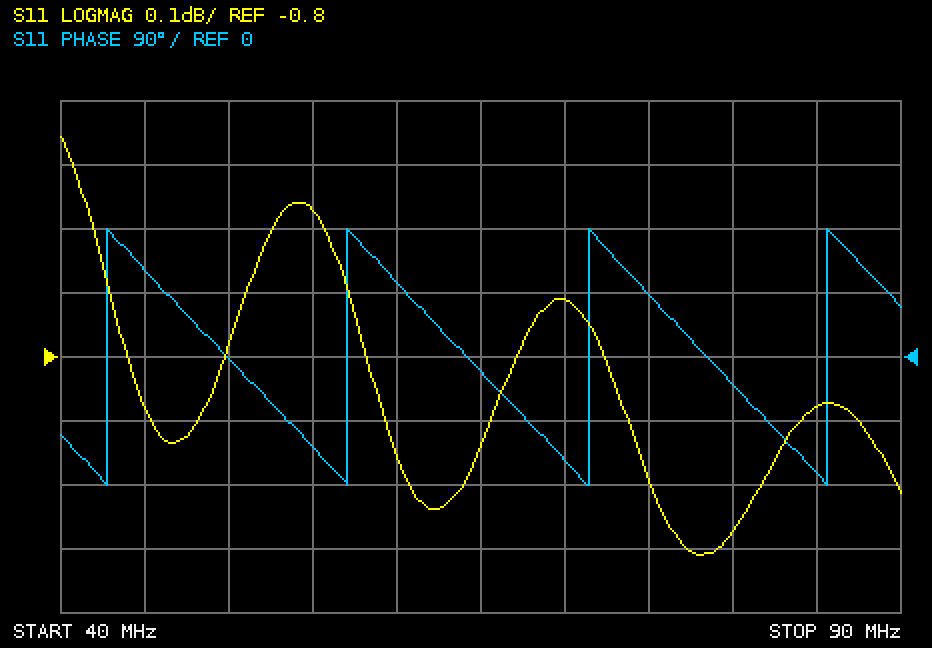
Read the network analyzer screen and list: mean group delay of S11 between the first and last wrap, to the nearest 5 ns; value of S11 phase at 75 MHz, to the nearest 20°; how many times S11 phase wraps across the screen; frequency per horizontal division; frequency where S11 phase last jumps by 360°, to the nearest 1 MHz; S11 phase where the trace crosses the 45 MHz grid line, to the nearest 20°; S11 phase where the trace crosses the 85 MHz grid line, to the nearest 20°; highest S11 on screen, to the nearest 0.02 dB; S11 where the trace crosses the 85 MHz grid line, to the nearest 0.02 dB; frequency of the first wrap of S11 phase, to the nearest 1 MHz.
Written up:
70 ns
80°
4
5 MHz
86 MHz
120°
-160°
-0.46 dB
-0.88 dB
43 MHz
